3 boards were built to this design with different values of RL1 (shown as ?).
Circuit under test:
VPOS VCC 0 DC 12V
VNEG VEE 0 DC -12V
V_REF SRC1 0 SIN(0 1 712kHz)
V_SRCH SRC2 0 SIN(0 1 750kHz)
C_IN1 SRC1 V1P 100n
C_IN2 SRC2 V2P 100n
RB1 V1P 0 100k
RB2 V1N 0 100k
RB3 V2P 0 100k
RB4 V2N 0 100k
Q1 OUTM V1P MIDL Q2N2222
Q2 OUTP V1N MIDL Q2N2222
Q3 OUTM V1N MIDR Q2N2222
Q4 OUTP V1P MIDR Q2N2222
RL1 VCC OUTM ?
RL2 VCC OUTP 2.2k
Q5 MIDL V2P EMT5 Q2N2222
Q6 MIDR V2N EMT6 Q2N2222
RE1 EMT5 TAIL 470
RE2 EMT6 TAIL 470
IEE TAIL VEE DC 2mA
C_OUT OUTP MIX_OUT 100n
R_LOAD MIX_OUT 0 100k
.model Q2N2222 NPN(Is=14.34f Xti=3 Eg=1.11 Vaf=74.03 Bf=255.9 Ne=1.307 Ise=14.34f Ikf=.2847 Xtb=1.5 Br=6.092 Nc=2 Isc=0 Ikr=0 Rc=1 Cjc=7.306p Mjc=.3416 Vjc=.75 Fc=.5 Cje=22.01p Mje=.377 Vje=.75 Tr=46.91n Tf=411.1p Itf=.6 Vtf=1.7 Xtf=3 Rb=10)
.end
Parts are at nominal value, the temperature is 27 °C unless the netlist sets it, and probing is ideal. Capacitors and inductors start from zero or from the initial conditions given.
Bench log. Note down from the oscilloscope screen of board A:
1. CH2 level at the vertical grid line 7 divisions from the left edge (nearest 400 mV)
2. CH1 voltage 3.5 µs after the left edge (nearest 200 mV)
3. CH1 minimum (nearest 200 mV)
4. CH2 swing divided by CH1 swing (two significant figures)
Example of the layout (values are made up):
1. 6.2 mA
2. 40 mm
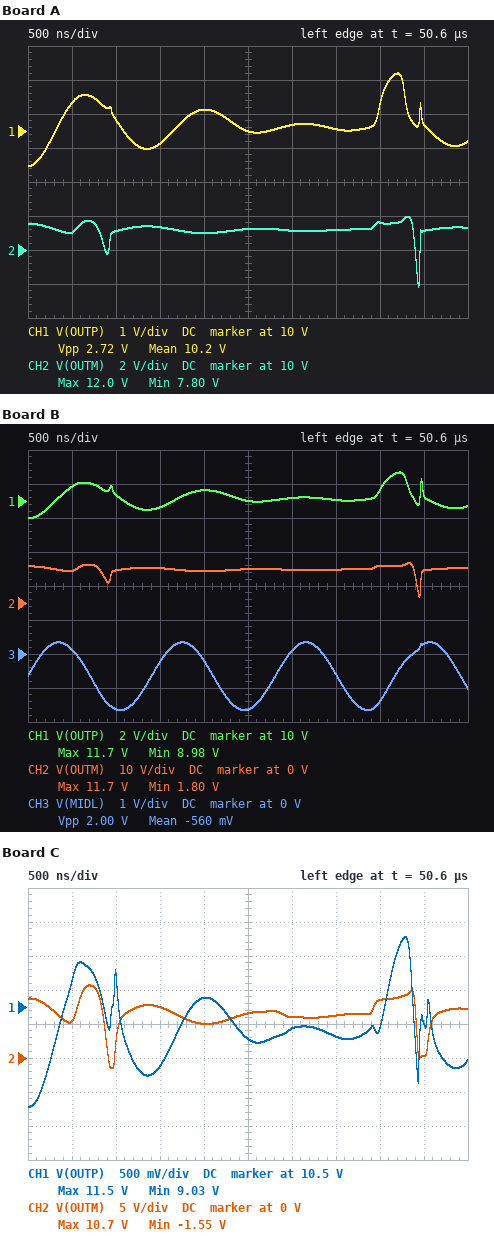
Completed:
1. 11.2 V
2. 10.0 V
3. 9.0 V
4. 1.5
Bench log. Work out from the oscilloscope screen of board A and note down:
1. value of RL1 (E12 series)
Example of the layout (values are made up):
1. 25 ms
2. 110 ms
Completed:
1. 680 Ω
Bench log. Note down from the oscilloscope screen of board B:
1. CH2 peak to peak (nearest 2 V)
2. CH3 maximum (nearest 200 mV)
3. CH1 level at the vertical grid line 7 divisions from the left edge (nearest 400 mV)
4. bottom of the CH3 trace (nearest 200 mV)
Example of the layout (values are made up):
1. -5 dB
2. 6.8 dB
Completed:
1. 10 V
2. 400 mV
3. 10.0 V
4. -1.6 V
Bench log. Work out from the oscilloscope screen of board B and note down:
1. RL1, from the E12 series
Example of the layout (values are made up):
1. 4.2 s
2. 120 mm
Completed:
1. 1.8 kΩ
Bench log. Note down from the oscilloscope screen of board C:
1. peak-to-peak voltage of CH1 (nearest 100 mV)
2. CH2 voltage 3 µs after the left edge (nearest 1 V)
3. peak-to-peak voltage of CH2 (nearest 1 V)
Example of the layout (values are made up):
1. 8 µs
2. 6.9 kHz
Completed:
1. 2.5 V
2. 6 V
3. 12 V
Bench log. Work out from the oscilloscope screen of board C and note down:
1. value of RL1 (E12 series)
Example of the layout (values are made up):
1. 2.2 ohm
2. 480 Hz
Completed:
1. 4.7 kΩ
